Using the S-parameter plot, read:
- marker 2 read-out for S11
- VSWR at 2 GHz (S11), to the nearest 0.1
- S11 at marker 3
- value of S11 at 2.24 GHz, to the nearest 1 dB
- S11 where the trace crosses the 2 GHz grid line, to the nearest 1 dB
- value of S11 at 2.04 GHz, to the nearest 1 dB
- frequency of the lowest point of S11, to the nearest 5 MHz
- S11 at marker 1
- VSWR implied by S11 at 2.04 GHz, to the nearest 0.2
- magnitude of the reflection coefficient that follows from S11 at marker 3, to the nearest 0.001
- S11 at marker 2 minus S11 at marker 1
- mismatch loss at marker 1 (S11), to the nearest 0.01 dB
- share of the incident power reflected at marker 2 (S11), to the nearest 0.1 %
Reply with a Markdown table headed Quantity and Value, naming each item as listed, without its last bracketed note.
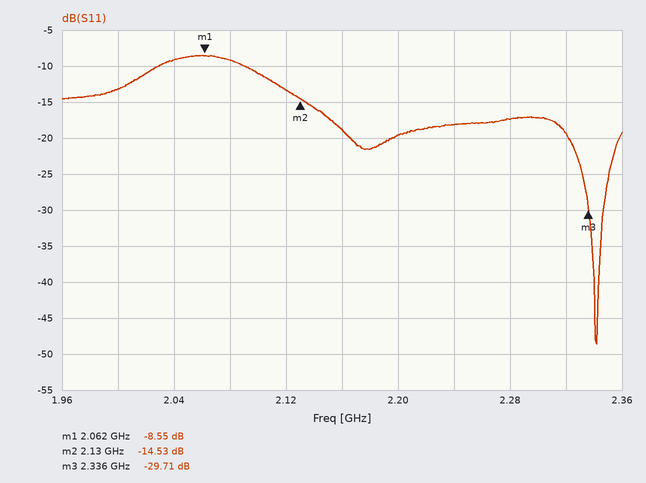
| Quantity | Value |
|---|---|
| marker 2 read-out for S11 | -14.53 dB |
| VSWR at 2 GHz (S11), to the nearest 0.1 | 1.6 |
| S11 at marker 3 | -29.71 dB |
| value of S11 at 2.24 GHz, to the nearest 1 dB | -18 dB |
| S11 where the trace crosses the 2 GHz grid line, to the nearest 1 dB | -13 dB |
| value of S11 at 2.04 GHz, to the nearest 1 dB | -9 dB |
| frequency of the lowest point of S11, to the nearest 5 MHz | 2.340 GHz |
| S11 at marker 1 | -8.55 dB |
| VSWR implied by S11 at 2.04 GHz, to the nearest 0.2 | 2.0 |
| magnitude of the reflection coefficient that follows from S11 at marker 3, to the nearest 0.001 | 0.033 |
| S11 at marker 2 minus S11 at marker 1 | -5.98 dB |
| mismatch loss at marker 1 (S11), to the nearest 0.01 dB | 0.65 dB |
| share of the incident power reflected at marker 2 (S11), to the nearest 0.1 % | 3.5 % |
